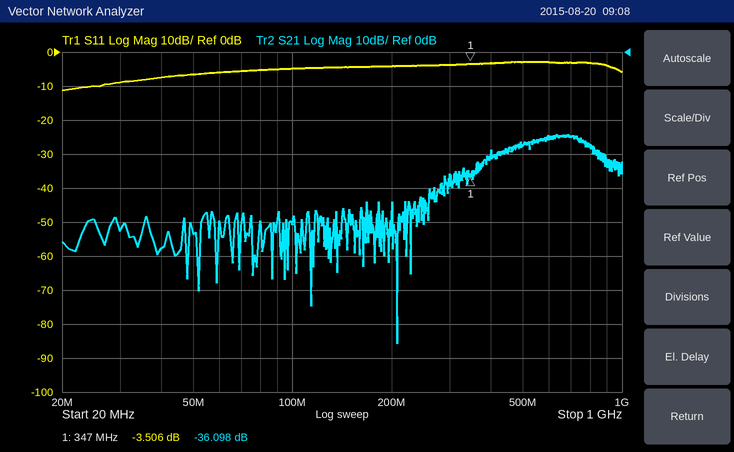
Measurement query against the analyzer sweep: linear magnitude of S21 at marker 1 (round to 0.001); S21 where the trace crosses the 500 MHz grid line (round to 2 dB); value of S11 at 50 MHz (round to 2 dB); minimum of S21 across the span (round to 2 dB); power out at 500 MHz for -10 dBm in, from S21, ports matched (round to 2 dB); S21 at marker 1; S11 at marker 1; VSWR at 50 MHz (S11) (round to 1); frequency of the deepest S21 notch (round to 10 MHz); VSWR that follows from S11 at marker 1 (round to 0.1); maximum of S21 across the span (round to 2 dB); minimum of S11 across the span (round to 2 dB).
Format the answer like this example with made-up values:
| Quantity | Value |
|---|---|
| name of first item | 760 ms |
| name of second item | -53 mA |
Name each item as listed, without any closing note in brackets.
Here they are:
| Quantity | Value |
|---|---|
| linear magnitude of S21 at marker 1 | 0.016 |
| S21 where the trace crosses the 500 MHz grid line | -28 dB |
| value of S11 at 50 MHz | -6 dB |
| minimum of S21 across the span | -86 dB |
| power out at 500 MHz for -10 dBm in, from S21, ports matched | -38 dBm |
| S21 at marker 1 | -36.098 dB |
| S11 at marker 1 | -3.506 dB |
| VSWR at 50 MHz (S11) | 3 |
| frequency of the deepest S21 notch | 210 MHz |
| VSWR that follows from S11 at marker 1 | 5.0 |
| maximum of S21 across the span | -24 dB |
| minimum of S11 across the span | -12 dB |
